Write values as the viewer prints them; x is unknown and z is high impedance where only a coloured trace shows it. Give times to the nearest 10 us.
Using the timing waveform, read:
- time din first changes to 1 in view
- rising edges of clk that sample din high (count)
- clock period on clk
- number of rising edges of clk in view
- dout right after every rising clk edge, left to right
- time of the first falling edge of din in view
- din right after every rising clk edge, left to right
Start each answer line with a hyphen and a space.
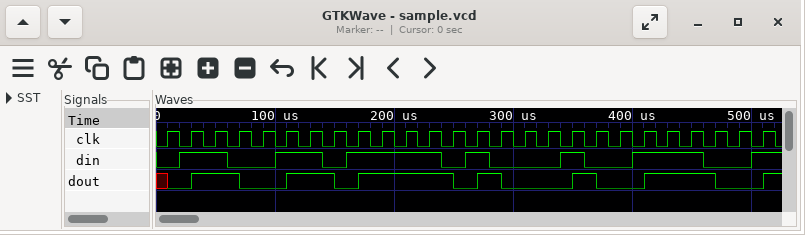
- 20 us
- 14
- 20 us
- 26
- 0 1 1 0 0 1 1 0 1 1 1 1 0 1 0 0 0 1 0 0 1 1 1 0 0 1
- 60 us
- 0 1 1 0 0 1 1 0 1 1 1 1 0 1 0 0 0 1 0 0 1 1 1 0 0 1
